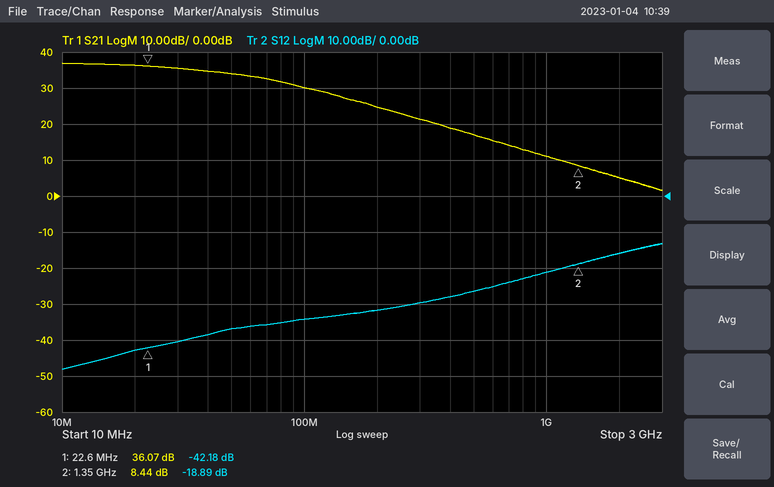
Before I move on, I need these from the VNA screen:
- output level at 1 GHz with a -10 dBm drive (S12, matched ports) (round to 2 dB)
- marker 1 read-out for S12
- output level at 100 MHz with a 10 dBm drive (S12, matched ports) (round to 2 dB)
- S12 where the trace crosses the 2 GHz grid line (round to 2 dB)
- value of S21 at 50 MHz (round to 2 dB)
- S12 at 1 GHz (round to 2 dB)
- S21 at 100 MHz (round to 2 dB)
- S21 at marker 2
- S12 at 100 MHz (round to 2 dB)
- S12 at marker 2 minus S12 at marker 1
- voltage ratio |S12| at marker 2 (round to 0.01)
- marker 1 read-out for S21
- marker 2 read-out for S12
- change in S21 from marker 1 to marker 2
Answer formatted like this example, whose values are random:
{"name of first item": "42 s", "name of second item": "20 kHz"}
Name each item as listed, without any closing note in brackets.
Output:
{"output level at 1 GHz with a -10 dBm drive (S12, matched ports)": "-32 dBm", "marker 1 read-out for S12": "-42.18 dB", "output level at 100 MHz with a 10 dBm drive (S12, matched ports)": "-24 dBm", "S12 where the trace crosses the 2 GHz grid line": "-16 dB", "value of S21 at 50 MHz": "34 dB", "S12 at 1 GHz": "-22 dB", "S21 at 100 MHz": "30 dB", "S21 at marker 2": "8.44 dB", "S12 at 100 MHz": "-34 dB", "S12 at marker 2 minus S12 at marker 1": "23.29 dB", "voltage ratio |S12| at marker 2": "0.11", "marker 1 read-out for S21": "36.07 dB", "marker 2 read-out for S12": "-18.89 dB", "change in S21 from marker 1 to marker 2": "-27.63 dB"}
